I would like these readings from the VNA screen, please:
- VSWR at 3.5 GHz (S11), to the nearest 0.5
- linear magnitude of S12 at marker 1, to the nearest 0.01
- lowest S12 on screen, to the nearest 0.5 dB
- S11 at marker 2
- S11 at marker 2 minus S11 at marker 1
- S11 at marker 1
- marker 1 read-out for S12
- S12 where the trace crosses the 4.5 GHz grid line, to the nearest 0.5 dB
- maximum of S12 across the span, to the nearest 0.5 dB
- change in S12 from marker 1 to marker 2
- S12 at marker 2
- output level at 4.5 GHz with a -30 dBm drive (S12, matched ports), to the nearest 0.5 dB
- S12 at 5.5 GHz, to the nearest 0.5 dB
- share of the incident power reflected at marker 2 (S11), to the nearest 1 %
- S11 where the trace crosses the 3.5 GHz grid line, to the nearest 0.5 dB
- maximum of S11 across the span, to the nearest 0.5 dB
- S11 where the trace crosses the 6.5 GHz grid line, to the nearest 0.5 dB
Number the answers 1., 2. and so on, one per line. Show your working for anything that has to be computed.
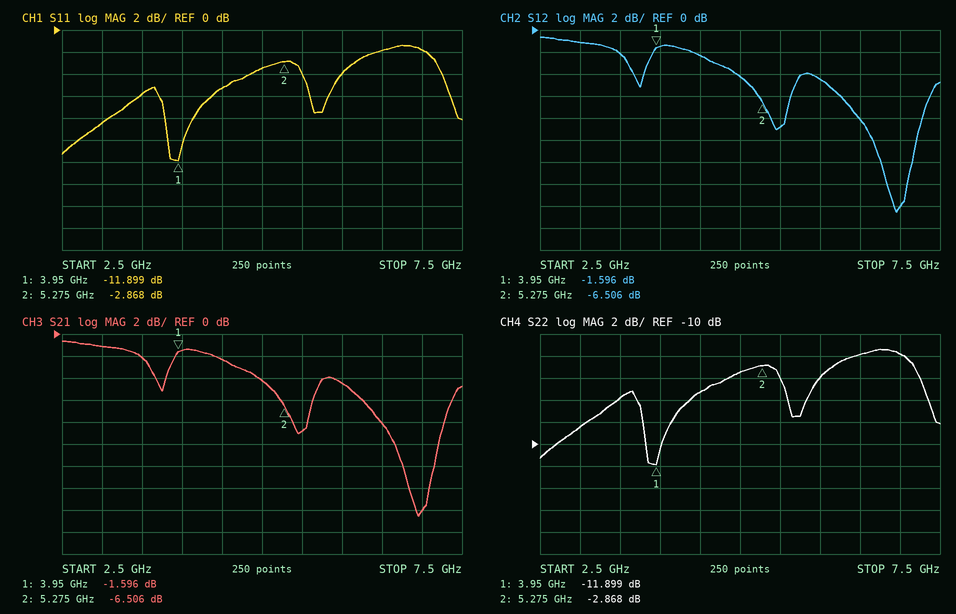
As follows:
1. |Γ| = 10^(-6/20) = 0.5012; VSWR = (1 + 0.5012)/(1 − 0.5012) ≈ 3.0
2. 10^(-1.596/20) ≈ 0.83
3. -16.5 dB
4. -2.868 dB
5. -2.868 − (-11.899) = 9.031 dB
6. -11.899 dB
7. -1.596 dB
8. -2.5 dB
9. -0.5 dB
10. -6.506 − (-1.596) = -4.910 dB
11. -6.506 dB
12. -30 dBm + (-2.5 dB) = -32.5 dBm
13. -9.0 dB
14. 10^(-2.868/10) ≈ 52 %
15. -6.0 dB
16. -1.5 dB
17. -2.0 dB
